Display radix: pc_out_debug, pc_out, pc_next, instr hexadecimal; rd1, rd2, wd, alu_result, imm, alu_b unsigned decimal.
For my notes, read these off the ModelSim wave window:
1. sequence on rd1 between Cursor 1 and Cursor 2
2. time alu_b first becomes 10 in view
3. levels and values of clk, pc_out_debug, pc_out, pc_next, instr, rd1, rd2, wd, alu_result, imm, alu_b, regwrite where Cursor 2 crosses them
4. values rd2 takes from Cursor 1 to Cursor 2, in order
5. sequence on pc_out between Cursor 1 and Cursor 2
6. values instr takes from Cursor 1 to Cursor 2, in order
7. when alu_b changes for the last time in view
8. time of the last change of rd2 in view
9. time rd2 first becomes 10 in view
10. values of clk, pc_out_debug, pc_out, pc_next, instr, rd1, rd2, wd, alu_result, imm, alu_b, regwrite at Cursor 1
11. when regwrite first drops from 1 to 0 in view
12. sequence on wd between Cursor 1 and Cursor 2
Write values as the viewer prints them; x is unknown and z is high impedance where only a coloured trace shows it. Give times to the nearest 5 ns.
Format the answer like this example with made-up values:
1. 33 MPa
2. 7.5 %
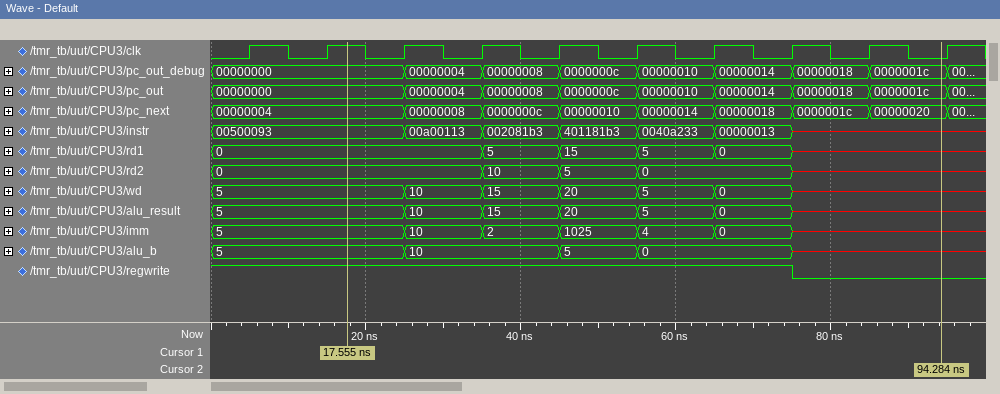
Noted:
1. 0, 5, 15, 5, 0, x
2. 25 ns
3. clk=0, pc_out_debug=0000001c, pc_out=0000001c, pc_next=00000020, instr=x, rd1=x, rd2=x, wd=x, alu_result=x, imm=x, alu_b=x, regwrite=0
4. 0, 10, 5, 0, x
5. 00000000, 00000004, 00000008, 0000000c, 00000010, 00000014, 00000018, 0000001c
6. 00500093, 00a00113, 002081b3, 401181b3, 0040a233, 00000013, x
7. 75 ns
8. 75 ns
9. 35 ns
10. clk=1, pc_out_debug=00000000, pc_out=00000000, pc_next=00000004, instr=00500093, rd1=0, rd2=0, wd=5, alu_result=5, imm=5, alu_b=5, regwrite=1
11. 75 ns
12. 5, 10, 15, 20, 5, 0, x
